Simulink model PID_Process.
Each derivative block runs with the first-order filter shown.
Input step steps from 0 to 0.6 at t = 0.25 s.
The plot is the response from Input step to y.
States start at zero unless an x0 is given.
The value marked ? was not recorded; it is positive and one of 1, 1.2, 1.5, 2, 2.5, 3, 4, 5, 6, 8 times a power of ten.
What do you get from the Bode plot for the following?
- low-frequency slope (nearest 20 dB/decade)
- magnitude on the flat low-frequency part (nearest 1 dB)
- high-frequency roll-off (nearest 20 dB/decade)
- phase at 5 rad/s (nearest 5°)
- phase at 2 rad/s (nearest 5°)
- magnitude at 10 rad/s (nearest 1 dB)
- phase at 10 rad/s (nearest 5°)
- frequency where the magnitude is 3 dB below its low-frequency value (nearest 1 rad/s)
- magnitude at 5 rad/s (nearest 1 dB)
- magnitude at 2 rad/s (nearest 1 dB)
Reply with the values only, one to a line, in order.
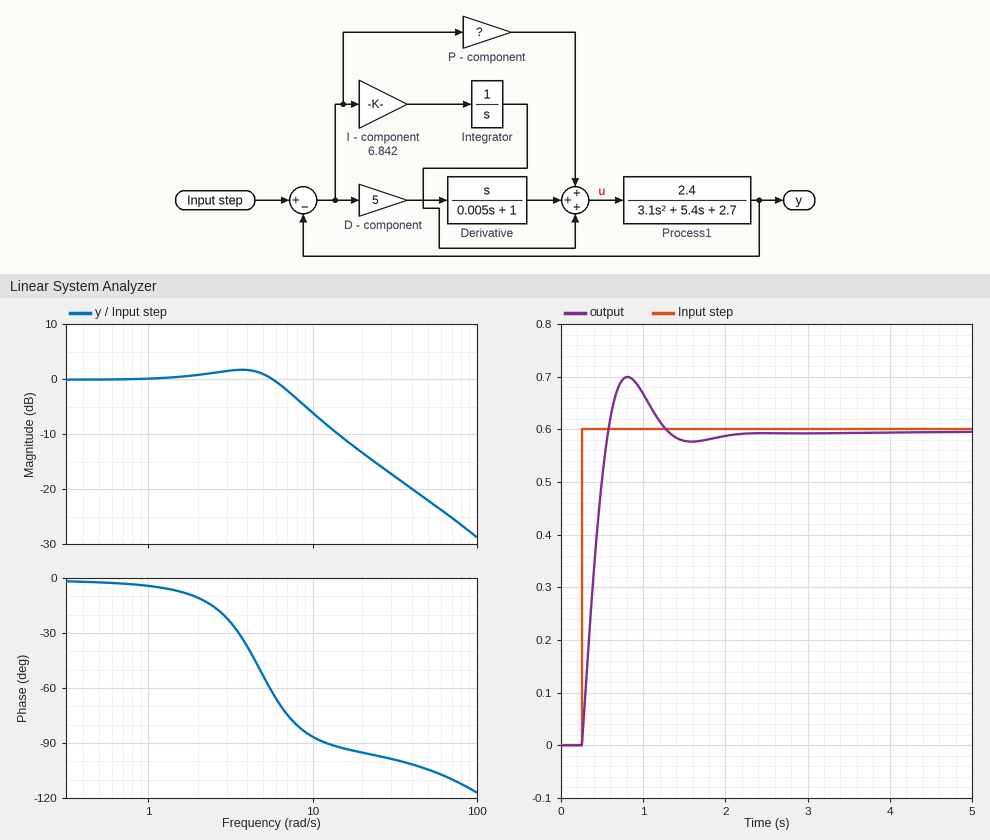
0 dB/decade
0 dB
-20 dB/decade
-55°
-10°
-6 dB
-85°
8 rad/s
1 dB
1 dB
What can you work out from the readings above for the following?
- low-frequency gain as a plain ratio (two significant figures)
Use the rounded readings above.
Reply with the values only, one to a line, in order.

1.0
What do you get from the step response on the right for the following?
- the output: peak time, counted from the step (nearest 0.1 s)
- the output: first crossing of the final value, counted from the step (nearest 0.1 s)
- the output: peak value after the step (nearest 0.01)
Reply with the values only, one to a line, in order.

0.6 s
0.3 s
0.70
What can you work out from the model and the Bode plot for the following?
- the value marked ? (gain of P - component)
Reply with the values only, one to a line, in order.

30
